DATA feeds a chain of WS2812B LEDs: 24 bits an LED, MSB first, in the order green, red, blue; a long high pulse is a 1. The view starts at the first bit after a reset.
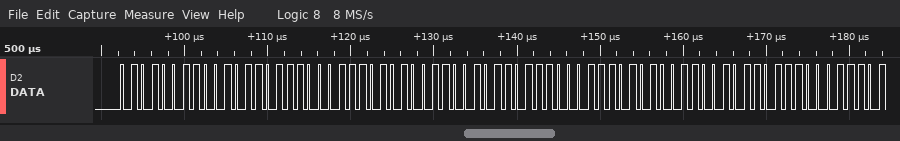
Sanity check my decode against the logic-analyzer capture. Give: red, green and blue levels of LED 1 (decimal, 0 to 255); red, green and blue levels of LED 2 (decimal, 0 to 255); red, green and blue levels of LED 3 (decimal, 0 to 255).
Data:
45, 83, 199
45, 83, 199
45, 83, 199
